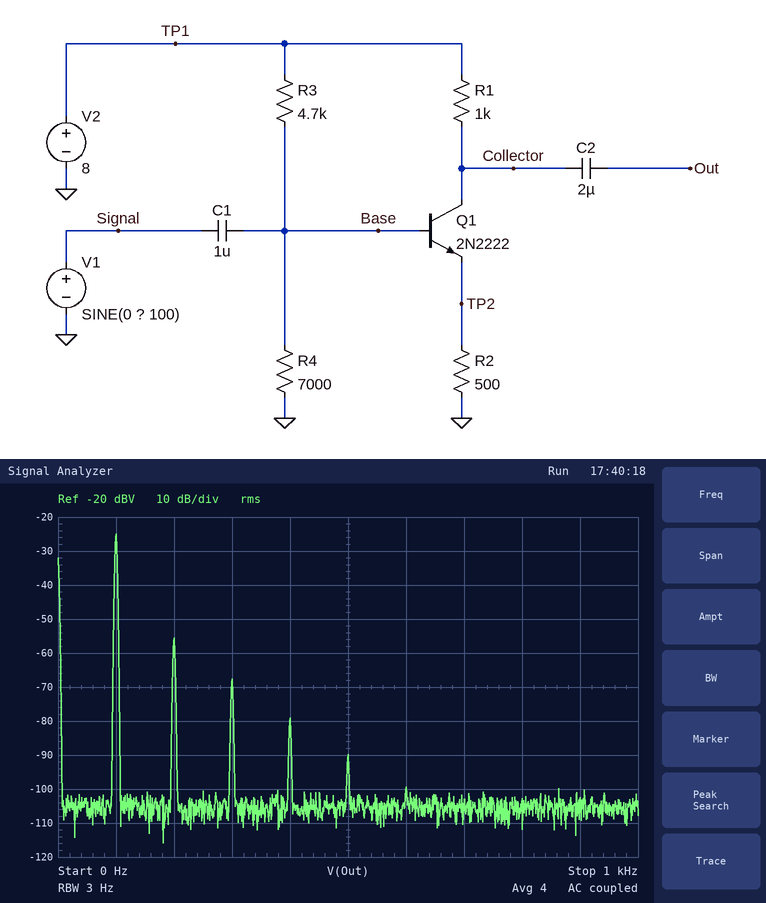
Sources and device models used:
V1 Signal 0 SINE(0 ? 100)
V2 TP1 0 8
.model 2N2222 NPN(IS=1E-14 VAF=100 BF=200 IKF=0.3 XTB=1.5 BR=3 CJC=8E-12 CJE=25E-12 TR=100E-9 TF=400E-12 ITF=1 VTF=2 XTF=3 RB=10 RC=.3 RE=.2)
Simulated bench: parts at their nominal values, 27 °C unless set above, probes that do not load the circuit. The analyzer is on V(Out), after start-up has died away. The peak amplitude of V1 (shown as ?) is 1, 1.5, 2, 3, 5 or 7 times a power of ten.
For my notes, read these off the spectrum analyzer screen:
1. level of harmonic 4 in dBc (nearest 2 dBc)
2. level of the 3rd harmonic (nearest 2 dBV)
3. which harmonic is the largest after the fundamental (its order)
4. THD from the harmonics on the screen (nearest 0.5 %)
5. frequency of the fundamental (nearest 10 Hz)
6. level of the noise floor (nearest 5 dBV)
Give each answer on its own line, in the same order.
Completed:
-54 dBc
-68 dBV
2
3.0 %
100 Hz
-105 dBV
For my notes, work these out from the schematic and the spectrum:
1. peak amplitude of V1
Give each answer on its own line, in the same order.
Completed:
500 mV
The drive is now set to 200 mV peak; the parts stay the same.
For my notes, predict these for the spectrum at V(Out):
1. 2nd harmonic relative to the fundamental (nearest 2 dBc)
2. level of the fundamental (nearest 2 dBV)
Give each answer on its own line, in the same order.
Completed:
-40 dBc
-32 dBV
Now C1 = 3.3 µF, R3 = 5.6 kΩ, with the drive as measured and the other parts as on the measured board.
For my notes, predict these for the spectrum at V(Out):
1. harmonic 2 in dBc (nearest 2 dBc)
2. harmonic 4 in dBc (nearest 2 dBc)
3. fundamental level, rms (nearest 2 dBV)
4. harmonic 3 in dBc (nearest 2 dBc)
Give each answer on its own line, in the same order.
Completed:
0 dBc
-14 dBc
-16 dBV
-18 dBc
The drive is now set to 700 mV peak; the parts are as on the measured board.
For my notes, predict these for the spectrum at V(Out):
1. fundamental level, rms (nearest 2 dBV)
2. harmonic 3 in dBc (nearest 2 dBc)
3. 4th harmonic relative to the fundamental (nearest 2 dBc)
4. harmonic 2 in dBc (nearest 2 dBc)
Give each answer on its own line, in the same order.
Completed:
-22 dBV
-32 dBc
-40 dBc
-24 dBc
